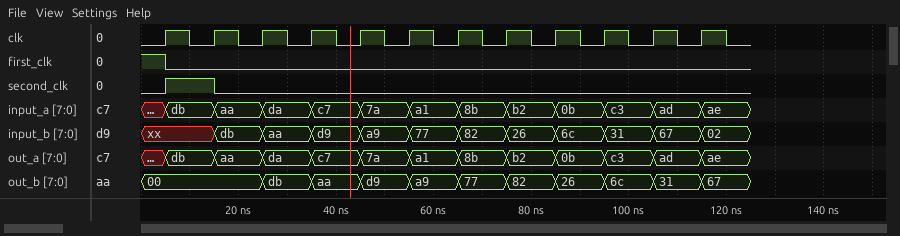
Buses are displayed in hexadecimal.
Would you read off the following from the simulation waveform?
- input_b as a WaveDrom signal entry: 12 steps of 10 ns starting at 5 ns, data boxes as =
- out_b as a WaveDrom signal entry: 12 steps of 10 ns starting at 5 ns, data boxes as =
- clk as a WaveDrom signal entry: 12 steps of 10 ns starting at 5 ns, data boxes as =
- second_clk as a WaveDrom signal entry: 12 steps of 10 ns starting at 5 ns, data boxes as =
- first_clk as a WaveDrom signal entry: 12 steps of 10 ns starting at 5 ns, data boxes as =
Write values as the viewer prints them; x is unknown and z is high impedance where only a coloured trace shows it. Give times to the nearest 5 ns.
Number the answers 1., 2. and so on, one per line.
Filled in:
1. {name: 'input_b', wave: 'x===========', data: 'db aa d9 a9 77 82 26 6c 31 67 02'}
2. {name: 'out_b', wave: '=.==========', data: '00 db aa d9 a9 77 82 26 6c 31 67'}
3. {name: 'clk', wave: 'p...........'}
4. {name: 'second_clk', wave: '10..........'}
5. {name: 'first_clk', wave: '0...........'}
